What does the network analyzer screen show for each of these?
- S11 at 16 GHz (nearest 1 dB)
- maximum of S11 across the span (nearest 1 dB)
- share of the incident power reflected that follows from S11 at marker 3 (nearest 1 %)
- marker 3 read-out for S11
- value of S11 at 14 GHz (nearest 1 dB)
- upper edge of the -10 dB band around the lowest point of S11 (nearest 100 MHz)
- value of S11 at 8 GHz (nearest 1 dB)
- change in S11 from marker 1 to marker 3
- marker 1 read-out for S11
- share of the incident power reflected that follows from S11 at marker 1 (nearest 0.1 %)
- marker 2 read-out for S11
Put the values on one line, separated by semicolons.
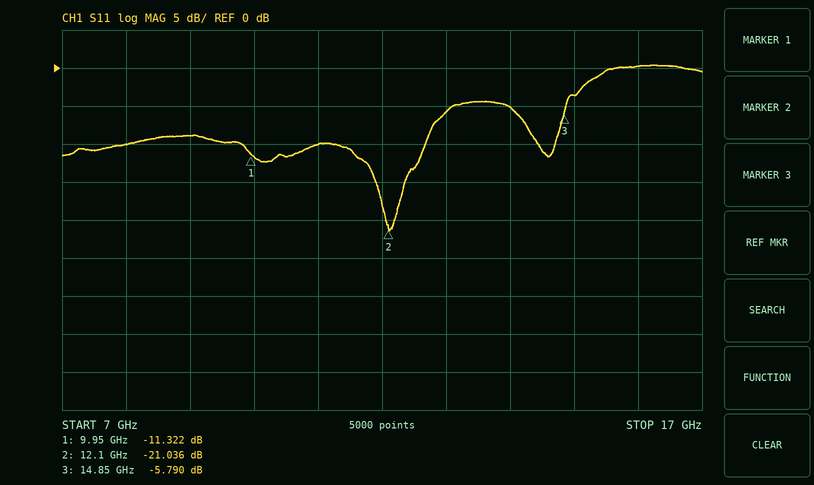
0 dB; 0 dB; 26 %; -5.790 dB; -5 dB; 12.7 GHz; -10 dB; 5.532 dB; -11.322 dB; 7.4 %; -21.036 dB
